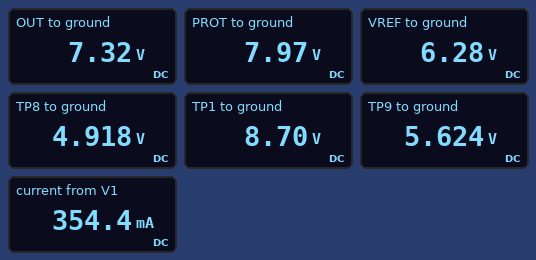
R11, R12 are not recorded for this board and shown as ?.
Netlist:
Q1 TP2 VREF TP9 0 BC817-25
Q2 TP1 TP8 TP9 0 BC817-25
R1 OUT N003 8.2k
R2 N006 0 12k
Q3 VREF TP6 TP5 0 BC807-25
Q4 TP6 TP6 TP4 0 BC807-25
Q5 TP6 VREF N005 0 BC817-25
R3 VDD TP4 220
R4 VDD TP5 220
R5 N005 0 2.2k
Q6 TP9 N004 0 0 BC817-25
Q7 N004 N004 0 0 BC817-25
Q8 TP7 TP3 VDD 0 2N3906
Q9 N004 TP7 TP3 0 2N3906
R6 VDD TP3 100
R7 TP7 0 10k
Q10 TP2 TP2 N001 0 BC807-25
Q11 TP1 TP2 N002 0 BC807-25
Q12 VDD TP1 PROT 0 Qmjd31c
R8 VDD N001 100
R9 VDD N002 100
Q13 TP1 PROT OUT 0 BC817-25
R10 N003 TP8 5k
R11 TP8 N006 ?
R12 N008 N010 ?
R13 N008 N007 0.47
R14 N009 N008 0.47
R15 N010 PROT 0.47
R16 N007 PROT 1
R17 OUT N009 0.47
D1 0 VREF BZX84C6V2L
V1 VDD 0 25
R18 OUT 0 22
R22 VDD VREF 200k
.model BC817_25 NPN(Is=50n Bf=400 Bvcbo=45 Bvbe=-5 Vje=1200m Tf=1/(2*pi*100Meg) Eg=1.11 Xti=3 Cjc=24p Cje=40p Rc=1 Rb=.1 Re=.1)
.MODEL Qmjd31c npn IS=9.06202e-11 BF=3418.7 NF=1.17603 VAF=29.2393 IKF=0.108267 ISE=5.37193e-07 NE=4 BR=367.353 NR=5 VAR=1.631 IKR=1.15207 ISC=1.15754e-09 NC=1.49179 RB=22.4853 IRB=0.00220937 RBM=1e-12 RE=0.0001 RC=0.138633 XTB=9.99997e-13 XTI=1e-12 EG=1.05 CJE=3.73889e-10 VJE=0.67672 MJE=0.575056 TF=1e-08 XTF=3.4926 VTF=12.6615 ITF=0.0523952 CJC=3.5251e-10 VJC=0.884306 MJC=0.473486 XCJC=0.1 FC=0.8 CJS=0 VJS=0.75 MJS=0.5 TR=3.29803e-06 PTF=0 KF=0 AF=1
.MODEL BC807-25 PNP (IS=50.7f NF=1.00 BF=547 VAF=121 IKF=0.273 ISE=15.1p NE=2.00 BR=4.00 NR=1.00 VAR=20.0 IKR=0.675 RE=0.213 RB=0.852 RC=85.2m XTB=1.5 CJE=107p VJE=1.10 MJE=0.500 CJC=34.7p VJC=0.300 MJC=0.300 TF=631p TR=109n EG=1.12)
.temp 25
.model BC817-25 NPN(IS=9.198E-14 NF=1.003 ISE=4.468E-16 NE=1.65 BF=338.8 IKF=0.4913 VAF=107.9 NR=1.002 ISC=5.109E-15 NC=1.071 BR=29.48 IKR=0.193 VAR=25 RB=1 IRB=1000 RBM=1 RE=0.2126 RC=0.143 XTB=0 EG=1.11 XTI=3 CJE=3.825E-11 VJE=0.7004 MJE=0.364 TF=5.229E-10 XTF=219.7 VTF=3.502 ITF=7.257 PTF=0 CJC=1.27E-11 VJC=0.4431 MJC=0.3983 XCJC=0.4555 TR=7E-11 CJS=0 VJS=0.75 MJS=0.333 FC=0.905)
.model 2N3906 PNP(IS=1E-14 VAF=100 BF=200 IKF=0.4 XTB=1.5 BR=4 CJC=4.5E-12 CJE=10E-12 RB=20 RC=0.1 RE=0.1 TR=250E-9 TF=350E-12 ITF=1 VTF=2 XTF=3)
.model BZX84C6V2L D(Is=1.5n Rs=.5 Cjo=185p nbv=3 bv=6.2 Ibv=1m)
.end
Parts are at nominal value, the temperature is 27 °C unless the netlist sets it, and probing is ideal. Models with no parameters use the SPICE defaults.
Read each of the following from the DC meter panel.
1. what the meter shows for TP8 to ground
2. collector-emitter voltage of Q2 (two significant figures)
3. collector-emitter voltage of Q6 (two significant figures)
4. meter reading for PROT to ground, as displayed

4.918 V
3.1 V
5.6 V
7.97 V
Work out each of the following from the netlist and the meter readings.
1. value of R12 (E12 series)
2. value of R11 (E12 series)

3.3 Ω
15 kΩ
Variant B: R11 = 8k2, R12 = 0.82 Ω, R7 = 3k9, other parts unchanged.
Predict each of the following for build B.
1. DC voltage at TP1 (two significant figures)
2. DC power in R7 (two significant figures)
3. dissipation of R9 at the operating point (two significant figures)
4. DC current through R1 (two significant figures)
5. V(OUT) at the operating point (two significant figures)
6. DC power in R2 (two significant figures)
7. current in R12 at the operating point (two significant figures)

10 V
140 mW
5.4 mW
270 µA
9.0 V
860 µW
210 mA
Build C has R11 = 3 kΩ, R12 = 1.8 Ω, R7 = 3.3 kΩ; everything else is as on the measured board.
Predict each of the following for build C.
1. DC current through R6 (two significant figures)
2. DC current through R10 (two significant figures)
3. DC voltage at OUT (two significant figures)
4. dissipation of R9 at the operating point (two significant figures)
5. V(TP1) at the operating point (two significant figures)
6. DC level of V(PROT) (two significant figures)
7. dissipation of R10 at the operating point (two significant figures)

7.1 mA
280 µA
8.0 V
5.4 mW
9.4 V
8.6 V
400 µW
